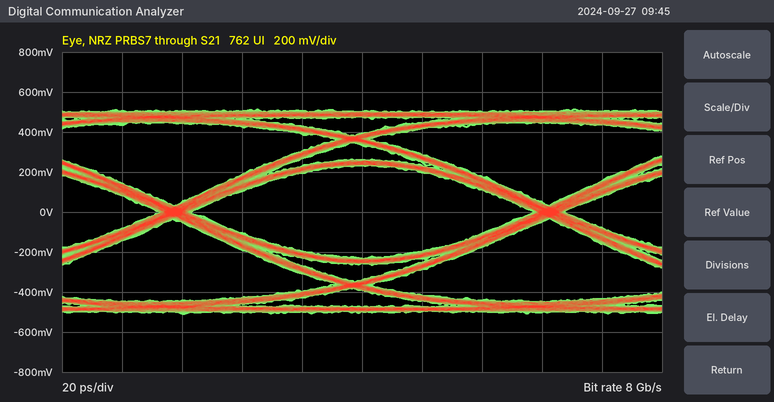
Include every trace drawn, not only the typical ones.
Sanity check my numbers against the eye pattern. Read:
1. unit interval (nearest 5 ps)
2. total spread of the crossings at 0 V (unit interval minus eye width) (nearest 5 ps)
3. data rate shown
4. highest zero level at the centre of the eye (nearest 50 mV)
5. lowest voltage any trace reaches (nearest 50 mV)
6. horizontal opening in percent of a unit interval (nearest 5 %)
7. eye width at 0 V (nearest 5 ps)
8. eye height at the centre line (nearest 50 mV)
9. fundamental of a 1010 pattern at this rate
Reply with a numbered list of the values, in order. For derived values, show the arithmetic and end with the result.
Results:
1. 125 ps
2. 10 ps
3. 8 Gb/s
4. -250 mV
5. -500 mV
6. 115 ps / 125 ps ≈ 92.0 %, so 90 % to the nearest 5 %
7. 115 ps
8. 450 mV
9. 4 GHz
